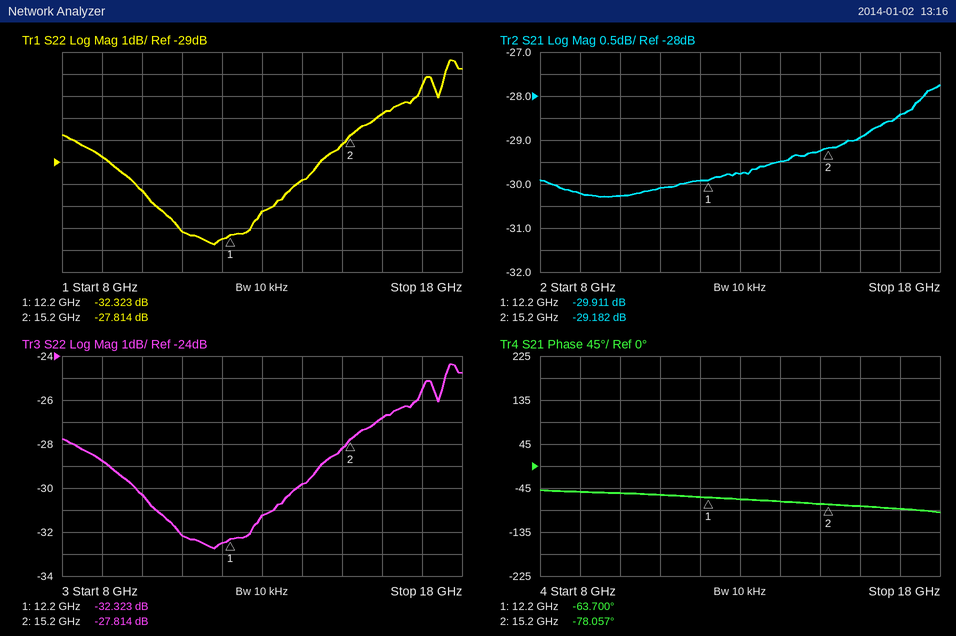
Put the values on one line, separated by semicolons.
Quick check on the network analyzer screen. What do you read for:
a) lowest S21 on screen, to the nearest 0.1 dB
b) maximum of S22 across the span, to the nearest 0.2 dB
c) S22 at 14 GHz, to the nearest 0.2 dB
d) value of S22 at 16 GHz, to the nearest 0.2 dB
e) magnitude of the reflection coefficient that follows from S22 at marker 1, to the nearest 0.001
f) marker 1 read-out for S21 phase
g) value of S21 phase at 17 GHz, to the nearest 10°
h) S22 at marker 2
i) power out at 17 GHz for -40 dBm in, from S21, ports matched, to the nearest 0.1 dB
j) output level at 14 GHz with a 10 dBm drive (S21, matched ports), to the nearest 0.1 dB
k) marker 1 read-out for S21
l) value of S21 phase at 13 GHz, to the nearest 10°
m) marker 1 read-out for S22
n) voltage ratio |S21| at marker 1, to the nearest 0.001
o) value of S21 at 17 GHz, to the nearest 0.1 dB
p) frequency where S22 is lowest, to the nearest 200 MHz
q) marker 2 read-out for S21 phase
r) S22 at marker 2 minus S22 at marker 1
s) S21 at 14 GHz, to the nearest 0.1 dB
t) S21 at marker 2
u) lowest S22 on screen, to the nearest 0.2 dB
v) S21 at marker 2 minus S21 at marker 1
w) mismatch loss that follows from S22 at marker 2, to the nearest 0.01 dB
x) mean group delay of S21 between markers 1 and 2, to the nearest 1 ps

-30.3 dB; -24.4 dB; -29.8 dB; -26.8 dB; 0.024; -63.700°; -90°; -27.814 dB; -68.4 dBm; -19.5 dBm; -29.911 dB; -70°; -32.323 dB; 0.032; -28.4 dB; 11.8 GHz; -78.057°; 4.509 dB; -29.5 dB; -29.182 dB; -32.8 dB; 0.729 dB; 0.01 dB; 13 ps
